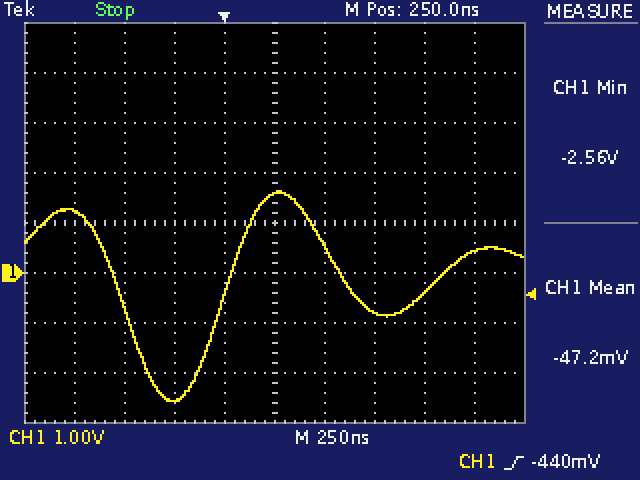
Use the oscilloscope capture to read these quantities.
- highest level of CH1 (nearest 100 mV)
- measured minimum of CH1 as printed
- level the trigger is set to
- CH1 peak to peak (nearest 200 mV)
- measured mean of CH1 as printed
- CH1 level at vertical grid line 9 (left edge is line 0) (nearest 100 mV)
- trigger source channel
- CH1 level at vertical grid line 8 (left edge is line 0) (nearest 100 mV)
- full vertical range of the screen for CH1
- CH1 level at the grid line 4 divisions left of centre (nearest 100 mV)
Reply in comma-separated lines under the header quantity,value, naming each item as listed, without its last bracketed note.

quantity,value
highest level of CH1,1.6 V
measured minimum of CH1 as printed,-2.56 V
level the trigger is set to,-440 mV
CH1 peak to peak,4.2 V
measured mean of CH1 as printed,-47.2 mV
CH1 level at vertical grid line 9 (left edge is line 0),400 mV
trigger source channel,CH1
CH1 level at vertical grid line 8 (left edge is line 0),-400 mV
full vertical range of the screen for CH1,8 V
CH1 level at the grid line 4 divisions left of centre,1.2 V
